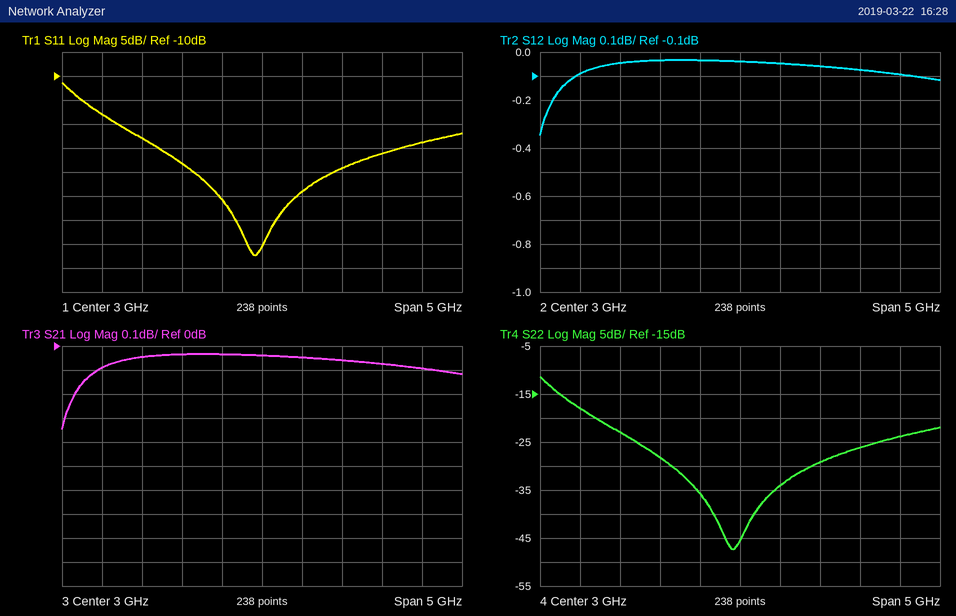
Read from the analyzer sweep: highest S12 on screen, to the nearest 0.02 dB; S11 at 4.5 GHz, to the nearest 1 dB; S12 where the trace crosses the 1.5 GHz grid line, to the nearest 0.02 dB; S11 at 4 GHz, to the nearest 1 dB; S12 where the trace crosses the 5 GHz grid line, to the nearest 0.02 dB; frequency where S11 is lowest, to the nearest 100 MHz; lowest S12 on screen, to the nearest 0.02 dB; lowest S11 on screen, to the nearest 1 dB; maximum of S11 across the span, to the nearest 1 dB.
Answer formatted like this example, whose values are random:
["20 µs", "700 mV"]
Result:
["-0.04 dB", "-26 dB", "-0.04 dB", "-29 dB", "-0.10 dB", "2.9 GHz", "-0.34 dB", "-47 dB", "-11 dB"]
